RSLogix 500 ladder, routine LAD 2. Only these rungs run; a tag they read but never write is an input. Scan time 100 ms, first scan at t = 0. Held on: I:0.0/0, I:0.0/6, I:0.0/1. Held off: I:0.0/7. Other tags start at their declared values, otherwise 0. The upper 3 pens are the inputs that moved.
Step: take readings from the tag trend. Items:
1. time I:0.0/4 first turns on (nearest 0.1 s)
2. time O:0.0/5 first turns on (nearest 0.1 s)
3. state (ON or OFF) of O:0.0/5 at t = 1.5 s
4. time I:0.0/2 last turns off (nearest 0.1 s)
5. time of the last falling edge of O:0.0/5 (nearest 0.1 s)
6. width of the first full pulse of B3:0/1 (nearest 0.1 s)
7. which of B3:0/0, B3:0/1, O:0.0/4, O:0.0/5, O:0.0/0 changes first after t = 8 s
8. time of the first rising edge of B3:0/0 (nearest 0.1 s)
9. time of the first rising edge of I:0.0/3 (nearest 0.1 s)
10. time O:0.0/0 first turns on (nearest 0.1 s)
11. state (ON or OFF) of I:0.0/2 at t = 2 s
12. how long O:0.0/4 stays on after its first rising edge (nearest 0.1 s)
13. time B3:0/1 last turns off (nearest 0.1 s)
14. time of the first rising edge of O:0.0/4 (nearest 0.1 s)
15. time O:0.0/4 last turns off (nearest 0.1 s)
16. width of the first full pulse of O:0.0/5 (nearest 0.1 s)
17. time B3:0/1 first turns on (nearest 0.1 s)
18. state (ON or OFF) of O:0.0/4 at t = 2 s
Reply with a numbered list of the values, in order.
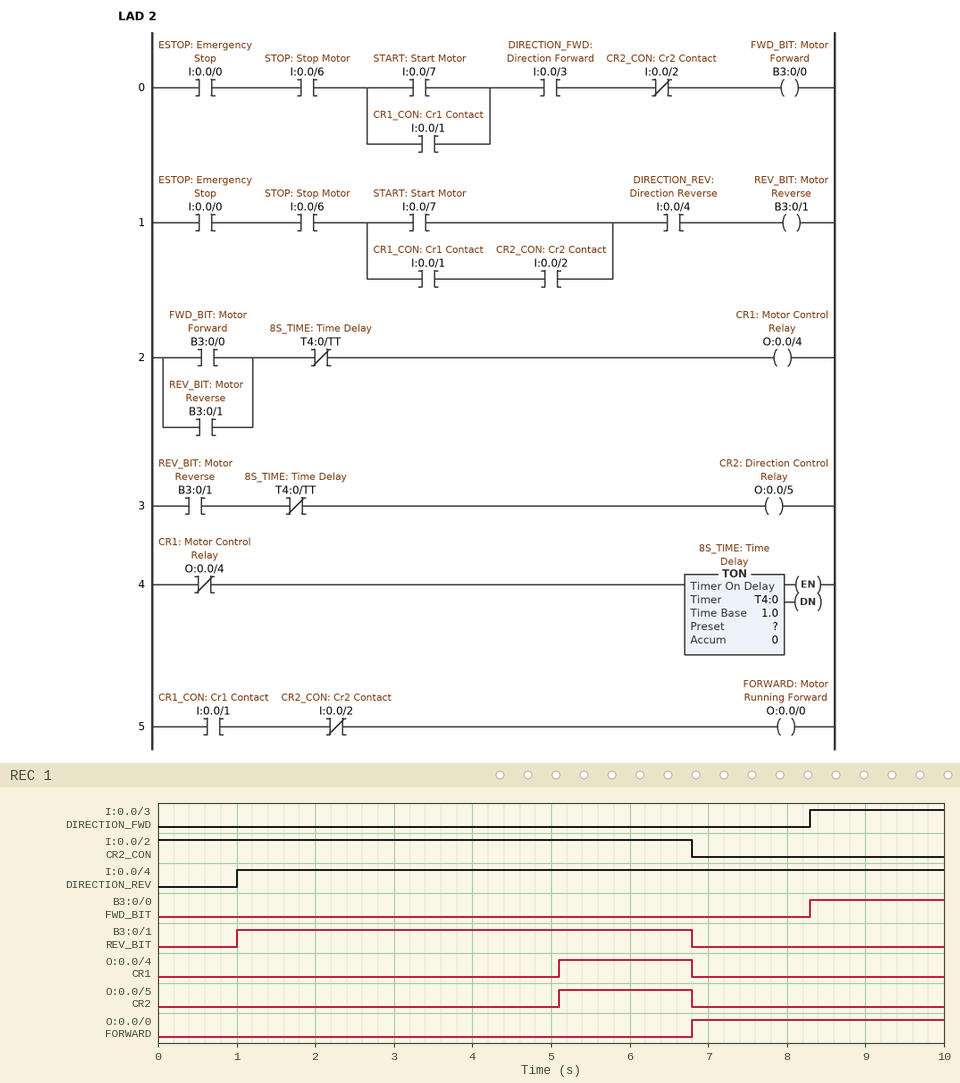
1. 1.0 s
2. 5.1 s
3. OFF
4. 6.8 s
5. 6.8 s
6. 5.8 s
7. B3:0/0
8. 8.3 s
9. 8.3 s
10. 6.8 s
11. ON
12. 1.7 s
13. 6.8 s
14. 5.1 s
15. 6.8 s
16. 1.7 s
17. 1.0 s
18. OFF
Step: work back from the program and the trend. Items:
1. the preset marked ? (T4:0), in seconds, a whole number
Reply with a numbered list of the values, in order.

1. 5 s
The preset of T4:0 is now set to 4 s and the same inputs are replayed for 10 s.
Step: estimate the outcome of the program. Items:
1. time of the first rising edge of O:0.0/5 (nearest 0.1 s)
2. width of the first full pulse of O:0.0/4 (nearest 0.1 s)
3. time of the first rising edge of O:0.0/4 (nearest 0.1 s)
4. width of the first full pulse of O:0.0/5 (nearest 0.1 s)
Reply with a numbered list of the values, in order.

1. 4.1 s
2. 2.7 s
3. 4.1 s
4. 2.7 s
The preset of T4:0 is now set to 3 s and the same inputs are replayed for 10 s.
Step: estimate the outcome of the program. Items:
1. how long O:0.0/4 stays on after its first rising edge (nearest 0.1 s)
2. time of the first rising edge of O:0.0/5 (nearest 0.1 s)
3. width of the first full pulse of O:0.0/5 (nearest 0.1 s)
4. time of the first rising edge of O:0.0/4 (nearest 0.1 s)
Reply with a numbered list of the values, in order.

1. 3.7 s
2. 3.1 s
3. 3.7 s
4. 3.1 s
